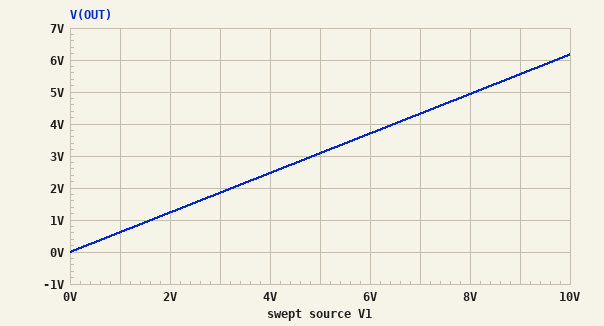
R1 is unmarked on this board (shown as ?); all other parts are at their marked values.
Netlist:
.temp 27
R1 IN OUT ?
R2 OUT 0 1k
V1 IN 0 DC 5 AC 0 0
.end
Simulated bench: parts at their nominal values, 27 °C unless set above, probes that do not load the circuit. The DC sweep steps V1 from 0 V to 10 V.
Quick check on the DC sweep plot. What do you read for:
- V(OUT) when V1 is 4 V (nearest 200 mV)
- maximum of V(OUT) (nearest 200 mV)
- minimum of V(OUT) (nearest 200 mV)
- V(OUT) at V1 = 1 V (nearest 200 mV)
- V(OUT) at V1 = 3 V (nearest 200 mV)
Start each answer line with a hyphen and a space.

- 2.4 V
- 6.2 V
- 0 V
- 600 mV
- 1.8 V
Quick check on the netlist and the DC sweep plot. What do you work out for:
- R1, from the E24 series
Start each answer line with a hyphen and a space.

- 620 Ω
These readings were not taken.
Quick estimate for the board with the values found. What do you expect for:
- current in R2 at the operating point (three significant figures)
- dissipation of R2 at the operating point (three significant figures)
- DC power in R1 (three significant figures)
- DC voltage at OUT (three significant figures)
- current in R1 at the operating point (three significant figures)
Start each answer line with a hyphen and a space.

- 3.09 mA
- 9.53 mW
- 5.91 mW
- 3.09 V
- 3.09 mA
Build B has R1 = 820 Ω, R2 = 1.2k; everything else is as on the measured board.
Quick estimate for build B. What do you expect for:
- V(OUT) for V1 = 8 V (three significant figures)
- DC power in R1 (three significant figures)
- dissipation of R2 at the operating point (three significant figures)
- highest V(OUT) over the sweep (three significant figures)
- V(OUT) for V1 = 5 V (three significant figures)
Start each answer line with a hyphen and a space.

- 4.75 V
- 5.02 mW
- 7.35 mW
- 5.94 V
- 2.97 V
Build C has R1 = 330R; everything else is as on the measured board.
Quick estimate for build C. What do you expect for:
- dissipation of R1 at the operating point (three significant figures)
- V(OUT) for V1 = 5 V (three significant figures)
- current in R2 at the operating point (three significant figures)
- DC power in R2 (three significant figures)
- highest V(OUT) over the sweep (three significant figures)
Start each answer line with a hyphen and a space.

- 4.66 mW
- 3.76 V
- 3.76 mA
- 14.1 mW
- 7.52 V
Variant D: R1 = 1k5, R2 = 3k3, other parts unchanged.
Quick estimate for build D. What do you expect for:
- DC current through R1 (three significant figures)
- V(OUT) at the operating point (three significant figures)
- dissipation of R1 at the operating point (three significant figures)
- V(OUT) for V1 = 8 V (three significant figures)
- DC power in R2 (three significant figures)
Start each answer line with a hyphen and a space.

- 1.04 mA
- 3.44 V
- 1.63 mW
- 5.50 V
- 3.58 mW
